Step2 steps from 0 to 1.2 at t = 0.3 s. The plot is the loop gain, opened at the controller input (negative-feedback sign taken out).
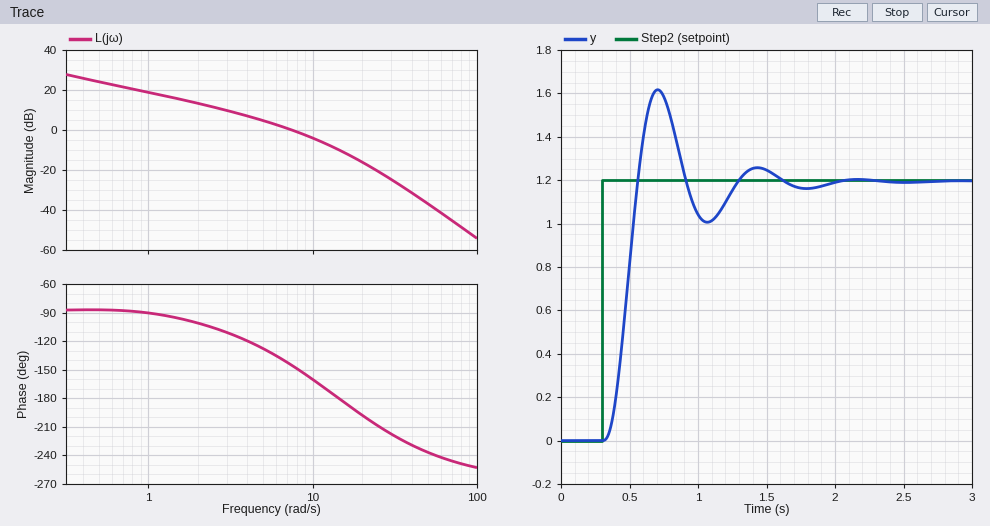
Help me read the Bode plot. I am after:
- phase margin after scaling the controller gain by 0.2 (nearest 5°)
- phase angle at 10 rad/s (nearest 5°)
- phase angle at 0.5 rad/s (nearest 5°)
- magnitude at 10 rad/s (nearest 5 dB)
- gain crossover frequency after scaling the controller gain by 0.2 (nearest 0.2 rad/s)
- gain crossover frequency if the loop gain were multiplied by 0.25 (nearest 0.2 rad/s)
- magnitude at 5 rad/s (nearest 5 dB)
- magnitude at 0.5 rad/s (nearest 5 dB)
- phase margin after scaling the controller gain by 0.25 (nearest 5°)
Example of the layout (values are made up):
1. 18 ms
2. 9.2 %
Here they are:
1. 80°
2. -160°
3. -85°
4. -5 dB
5. 1.8 rad/s
6. 2.4 rad/s
7. 5 dB
8. 25 dB
9. 75°
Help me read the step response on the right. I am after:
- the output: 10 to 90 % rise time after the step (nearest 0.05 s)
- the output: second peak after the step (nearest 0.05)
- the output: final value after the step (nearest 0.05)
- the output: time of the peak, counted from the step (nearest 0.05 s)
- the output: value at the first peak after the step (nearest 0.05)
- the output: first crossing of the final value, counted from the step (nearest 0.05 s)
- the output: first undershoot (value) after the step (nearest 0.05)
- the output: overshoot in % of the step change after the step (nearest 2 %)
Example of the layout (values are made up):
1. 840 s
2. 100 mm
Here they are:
1. 0.15 s
2. 1.25
3. 1.20
4. 0.40 s
5. 1.60
6. 0.25 s
7. 1.00
8. 34 %
